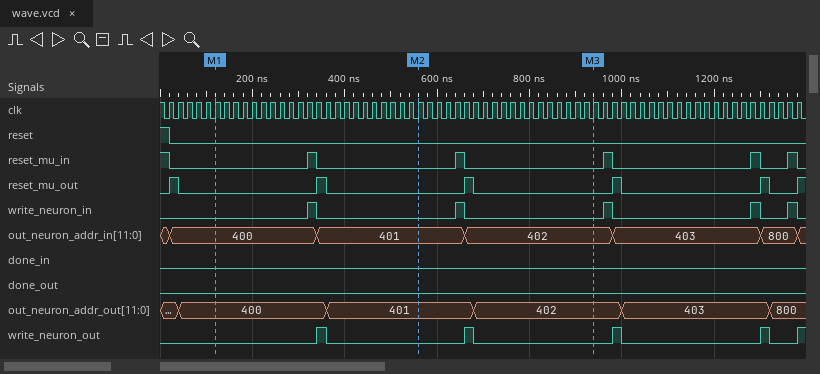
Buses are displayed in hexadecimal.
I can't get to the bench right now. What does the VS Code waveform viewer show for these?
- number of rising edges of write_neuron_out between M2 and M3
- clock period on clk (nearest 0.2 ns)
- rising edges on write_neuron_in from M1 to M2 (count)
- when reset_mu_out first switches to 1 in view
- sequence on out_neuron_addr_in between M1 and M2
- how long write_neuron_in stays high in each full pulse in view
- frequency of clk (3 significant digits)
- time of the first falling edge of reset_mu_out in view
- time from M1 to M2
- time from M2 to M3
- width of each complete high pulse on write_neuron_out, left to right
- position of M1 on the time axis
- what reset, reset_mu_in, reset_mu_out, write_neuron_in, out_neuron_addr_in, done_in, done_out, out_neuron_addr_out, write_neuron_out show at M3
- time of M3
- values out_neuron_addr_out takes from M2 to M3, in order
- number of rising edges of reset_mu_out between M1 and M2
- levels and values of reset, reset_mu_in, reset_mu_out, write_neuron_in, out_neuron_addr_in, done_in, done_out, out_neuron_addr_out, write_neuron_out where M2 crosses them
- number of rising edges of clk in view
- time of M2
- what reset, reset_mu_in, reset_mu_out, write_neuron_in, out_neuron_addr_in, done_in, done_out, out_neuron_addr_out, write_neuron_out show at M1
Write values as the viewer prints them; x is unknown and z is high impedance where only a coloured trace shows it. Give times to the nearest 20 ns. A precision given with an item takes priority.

1
20 ns
1
20 ns
400, 401
20 ns, 20 ns, 20 ns, 20 ns, 20 ns
50.0 MHz
40 ns
440 ns
380 ns
20 ns, 20 ns, 20 ns, 20 ns
120 ns
reset=0, reset_mu_in=0, reset_mu_out=0, write_neuron_in=0, out_neuron_addr_in=402, done_in=0, done_out=0, out_neuron_addr_out=402, write_neuron_out=0
940 ns
401, 402
1
reset=0, reset_mu_in=0, reset_mu_out=0, write_neuron_in=0, out_neuron_addr_in=401, done_in=0, done_out=0, out_neuron_addr_out=401, write_neuron_out=0
69
560 ns
reset=0, reset_mu_in=0, reset_mu_out=0, write_neuron_in=0, out_neuron_addr_in=400, done_in=0, done_out=0, out_neuron_addr_out=400, write_neuron_out=0
